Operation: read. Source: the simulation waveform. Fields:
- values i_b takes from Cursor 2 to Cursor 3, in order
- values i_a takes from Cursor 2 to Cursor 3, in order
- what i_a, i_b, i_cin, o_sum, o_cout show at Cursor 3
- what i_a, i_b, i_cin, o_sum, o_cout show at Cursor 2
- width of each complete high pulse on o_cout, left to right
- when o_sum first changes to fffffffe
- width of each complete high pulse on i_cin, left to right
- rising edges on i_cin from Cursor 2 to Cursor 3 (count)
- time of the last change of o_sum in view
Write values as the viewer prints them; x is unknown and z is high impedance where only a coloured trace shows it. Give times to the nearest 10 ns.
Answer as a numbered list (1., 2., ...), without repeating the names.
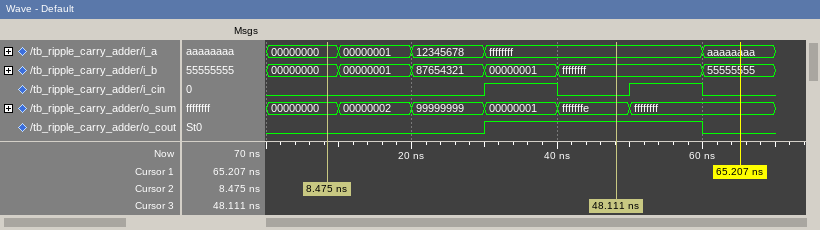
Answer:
1. 00000000, 00000001, 87654321, 00000001, ffffffff
2. 00000000, 00000001, 12345678, ffffffff
3. i_a=ffffffff, i_b=ffffffff, i_cin=0, o_sum=fffffffe, o_cout=1
4. i_a=00000000, i_b=00000000, i_cin=0, o_sum=00000000, o_cout=0
5. 30 ns
6. 40 ns
7. 10 ns, 10 ns
8. 1
9. 50 ns
